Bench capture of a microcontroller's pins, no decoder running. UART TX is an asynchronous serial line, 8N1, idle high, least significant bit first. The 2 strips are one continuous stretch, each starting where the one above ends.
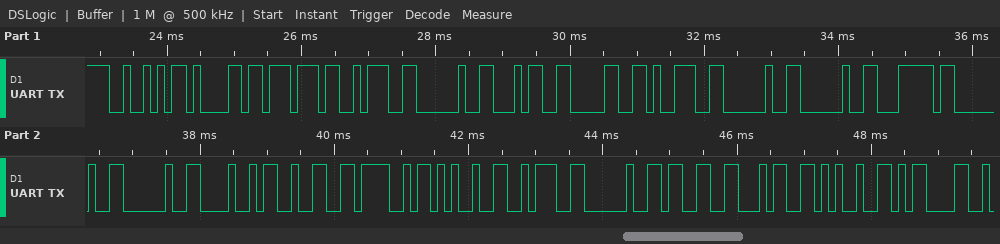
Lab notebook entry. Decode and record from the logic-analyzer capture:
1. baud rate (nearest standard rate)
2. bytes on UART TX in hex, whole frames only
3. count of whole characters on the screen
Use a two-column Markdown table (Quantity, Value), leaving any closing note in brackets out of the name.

| Quantity | Value |
|---|---|
| baud rate | 9600 baud |
| bytes on UART TX in hex, whole frames only | 52 61 77 3A 20 34 30 39 20 20 7C 20 20 48 32 4F 25 3A 20 33 34 25 0D |
| count of whole characters on the screen | 23 |
